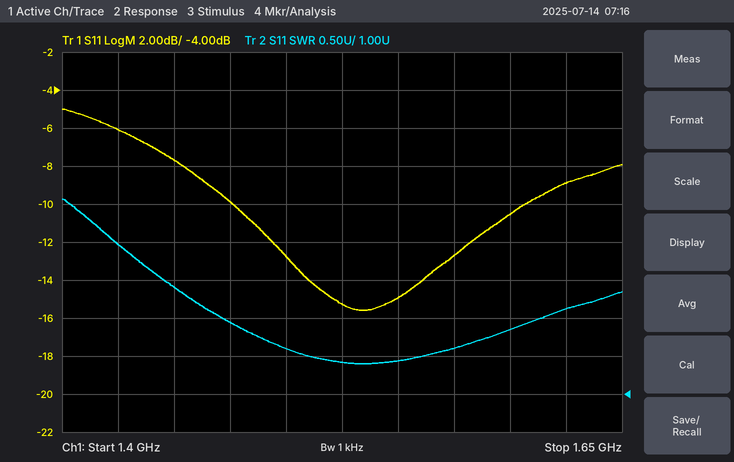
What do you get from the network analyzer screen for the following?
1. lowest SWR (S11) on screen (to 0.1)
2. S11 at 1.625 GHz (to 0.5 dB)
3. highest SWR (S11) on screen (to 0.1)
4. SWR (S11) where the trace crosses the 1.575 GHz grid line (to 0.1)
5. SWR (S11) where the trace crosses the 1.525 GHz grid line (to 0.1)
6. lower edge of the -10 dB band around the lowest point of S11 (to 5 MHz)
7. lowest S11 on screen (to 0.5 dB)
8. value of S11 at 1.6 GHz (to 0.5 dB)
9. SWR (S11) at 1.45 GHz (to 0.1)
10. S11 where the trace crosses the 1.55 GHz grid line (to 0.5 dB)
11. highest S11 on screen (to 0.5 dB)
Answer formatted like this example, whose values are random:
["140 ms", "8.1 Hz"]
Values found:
["1.4", "-9.0 dB", "3.6", "1.6", "1.4", "1.475 GHz", "-15.5 dB", "-10.5 dB", "2.4", "-15.0 dB", "-5.0 dB"]
